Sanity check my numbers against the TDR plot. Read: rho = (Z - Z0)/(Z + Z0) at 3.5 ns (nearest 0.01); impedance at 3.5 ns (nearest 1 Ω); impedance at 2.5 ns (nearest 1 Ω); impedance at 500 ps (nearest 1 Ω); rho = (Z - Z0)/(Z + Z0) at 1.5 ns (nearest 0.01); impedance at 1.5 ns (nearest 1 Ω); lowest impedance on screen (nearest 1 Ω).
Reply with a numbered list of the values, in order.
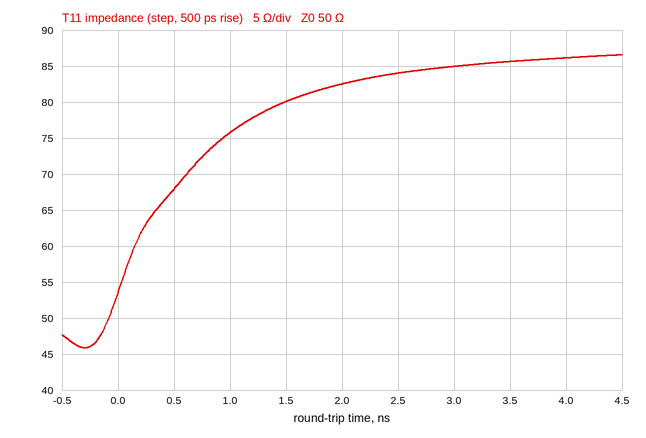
1. +0.26
2. 86 Ω
3. 84 Ω
4. 68 Ω
5. +0.23
6. 80 Ω
7. 46 Ω
